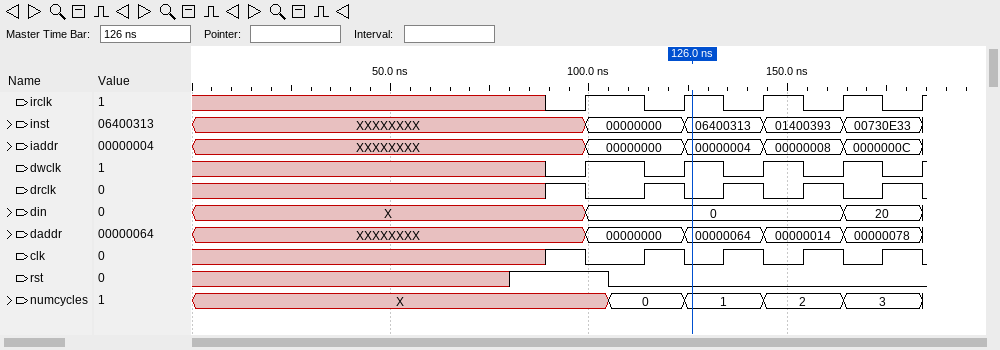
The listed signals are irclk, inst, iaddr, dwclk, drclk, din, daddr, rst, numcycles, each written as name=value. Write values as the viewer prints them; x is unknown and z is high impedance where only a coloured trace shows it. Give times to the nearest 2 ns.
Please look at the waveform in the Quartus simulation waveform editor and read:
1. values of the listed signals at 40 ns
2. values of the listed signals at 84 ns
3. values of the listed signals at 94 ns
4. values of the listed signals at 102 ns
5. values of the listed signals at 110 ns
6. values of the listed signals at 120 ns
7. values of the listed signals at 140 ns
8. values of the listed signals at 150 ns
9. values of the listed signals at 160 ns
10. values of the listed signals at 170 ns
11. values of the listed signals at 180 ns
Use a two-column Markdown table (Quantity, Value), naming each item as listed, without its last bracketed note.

| Quantity | Value |
|---|---|
| values of the listed signals at 40 ns | irclk=x, inst=XXXXXXXX, iaddr=XXXXXXXX, dwclk=x, drclk=x, din=X, daddr=XXXXXXXX, rst=x, numcycles=X |
| values of the listed signals at 84 ns | irclk=x, inst=XXXXXXXX, iaddr=XXXXXXXX, dwclk=x, drclk=x, din=X, daddr=XXXXXXXX, rst=1, numcycles=X |
| values of the listed signals at 94 ns | irclk=0, inst=XXXXXXXX, iaddr=XXXXXXXX, dwclk=0, drclk=1, din=X, daddr=XXXXXXXX, rst=1, numcycles=X |
| values of the listed signals at 102 ns | irclk=1, inst=00000000, iaddr=00000000, dwclk=1, drclk=0, din=0, daddr=00000000, rst=1, numcycles=X |
| values of the listed signals at 110 ns | irclk=1, inst=00000000, iaddr=00000000, dwclk=1, drclk=0, din=0, daddr=00000000, rst=0, numcycles=0 |
| values of the listed signals at 120 ns | irclk=0, inst=00000000, iaddr=00000000, dwclk=0, drclk=1, din=0, daddr=00000000, rst=0, numcycles=0 |
| values of the listed signals at 140 ns | irclk=0, inst=06400313, iaddr=00000004, dwclk=0, drclk=1, din=0, daddr=00000064, rst=0, numcycles=1 |
| values of the listed signals at 150 ns | irclk=1, inst=01400393, iaddr=00000008, dwclk=1, drclk=0, din=0, daddr=00000014, rst=0, numcycles=2 |
| values of the listed signals at 160 ns | irclk=0, inst=01400393, iaddr=00000008, dwclk=0, drclk=1, din=0, daddr=00000014, rst=0, numcycles=2 |
| values of the listed signals at 170 ns | irclk=1, inst=00730E33, iaddr=0000000C, dwclk=1, drclk=0, din=20, daddr=00000078, rst=0, numcycles=3 |
| values of the listed signals at 180 ns | irclk=0, inst=00730E33, iaddr=0000000C, dwclk=0, drclk=1, din=20, daddr=00000078, rst=0, numcycles=3 |
